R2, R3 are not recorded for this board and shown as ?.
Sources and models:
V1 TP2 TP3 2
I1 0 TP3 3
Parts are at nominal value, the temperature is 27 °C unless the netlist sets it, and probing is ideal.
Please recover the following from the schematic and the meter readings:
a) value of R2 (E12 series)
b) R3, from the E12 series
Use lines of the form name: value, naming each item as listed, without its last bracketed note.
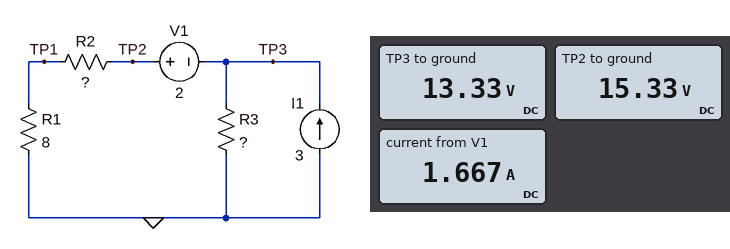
value of R2: 1.2 Ω
R3, from the E12 series: 10 Ω
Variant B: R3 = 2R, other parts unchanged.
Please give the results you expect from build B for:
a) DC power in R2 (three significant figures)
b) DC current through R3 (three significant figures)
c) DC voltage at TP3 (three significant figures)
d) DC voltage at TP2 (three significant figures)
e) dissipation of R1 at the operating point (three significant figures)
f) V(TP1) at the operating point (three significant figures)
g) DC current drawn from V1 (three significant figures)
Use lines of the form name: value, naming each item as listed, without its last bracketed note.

DC power in R2: 612 mW
DC current through R3: 2.29 A
DC voltage at TP3: 4.57 V
DC voltage at TP2: 6.57 V
dissipation of R1 at the operating point: 4.08 W
V(TP1) at the operating point: 5.71 V
DC current drawn from V1: 714 mA
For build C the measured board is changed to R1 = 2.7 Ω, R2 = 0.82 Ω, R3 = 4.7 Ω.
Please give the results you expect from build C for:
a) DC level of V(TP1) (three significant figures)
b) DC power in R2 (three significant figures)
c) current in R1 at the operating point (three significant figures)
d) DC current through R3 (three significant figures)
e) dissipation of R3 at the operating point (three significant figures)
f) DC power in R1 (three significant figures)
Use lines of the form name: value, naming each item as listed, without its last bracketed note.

DC level of V(TP1): 5.29 V
DC power in R2: 3.15 W
current in R1 at the operating point: 1.96 A
DC current through R3: 1.04 A
dissipation of R3 at the operating point: 5.10 W
DC power in R1: 10.4 W
